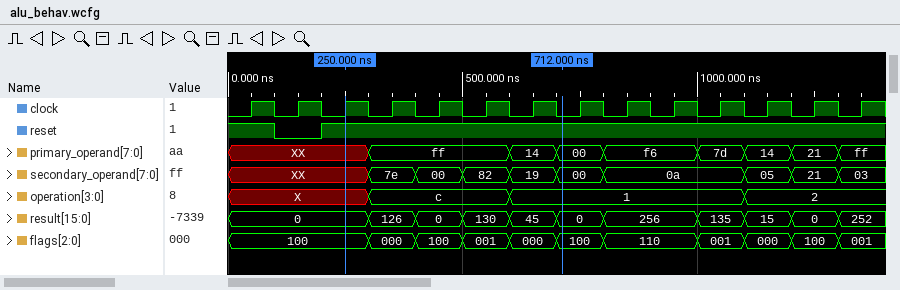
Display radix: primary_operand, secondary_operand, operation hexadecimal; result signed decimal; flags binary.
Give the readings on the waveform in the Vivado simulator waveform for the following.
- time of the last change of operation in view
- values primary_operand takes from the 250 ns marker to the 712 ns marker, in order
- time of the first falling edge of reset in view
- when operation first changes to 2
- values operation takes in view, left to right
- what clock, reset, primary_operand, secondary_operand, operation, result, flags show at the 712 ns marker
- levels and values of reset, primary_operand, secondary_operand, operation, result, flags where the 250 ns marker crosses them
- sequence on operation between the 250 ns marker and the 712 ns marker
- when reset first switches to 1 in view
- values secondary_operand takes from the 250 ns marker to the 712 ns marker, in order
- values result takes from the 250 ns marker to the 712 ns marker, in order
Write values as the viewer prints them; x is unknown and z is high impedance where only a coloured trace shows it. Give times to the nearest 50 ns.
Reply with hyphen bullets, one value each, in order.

- 1100 ns
- XX, ff, 14, 00
- 100 ns
- 1100 ns
- X, c, 1, 2
- clock=0, reset=1, primary_operand=00, secondary_operand=00, operation=1, result=0, flags=100
- reset=1, primary_operand=XX, secondary_operand=XX, operation=X, result=0, flags=100
- X, c, 1
- 200 ns
- XX, 7e, 00, 82, 19, 00
- 0, 126, 0, 130, 45, 0
